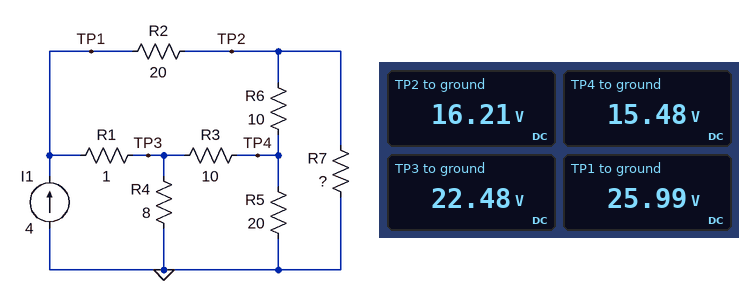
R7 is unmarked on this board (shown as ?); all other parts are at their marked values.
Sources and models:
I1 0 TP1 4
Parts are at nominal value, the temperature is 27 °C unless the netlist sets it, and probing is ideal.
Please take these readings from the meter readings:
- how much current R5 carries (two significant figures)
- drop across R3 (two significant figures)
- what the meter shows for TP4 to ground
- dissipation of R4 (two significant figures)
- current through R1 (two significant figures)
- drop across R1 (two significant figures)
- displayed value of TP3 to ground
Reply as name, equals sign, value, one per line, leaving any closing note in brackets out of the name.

how much current R5 carries = 770 mA
drop across R3 = 7.0 V
what the meter shows for TP4 to ground = 15.48 V
dissipation of R4 = 63 W
current through R1 = 3.5 A
drop across R1 = 3.5 V
displayed value of TP3 to ground = 22.48 V
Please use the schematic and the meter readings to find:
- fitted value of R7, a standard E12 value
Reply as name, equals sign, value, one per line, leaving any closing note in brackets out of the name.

fitted value of R7, a standard E12 value = 39 Ω
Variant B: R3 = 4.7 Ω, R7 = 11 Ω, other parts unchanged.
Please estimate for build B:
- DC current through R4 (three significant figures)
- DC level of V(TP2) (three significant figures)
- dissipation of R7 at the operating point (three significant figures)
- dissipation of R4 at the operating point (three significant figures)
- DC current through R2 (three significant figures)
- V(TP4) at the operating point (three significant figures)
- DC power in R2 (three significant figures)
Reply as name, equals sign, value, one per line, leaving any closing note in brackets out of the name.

DC current through R4 = 2.36 A
DC level of V(TP2) = 10.4 V
dissipation of R7 at the operating point = 9.84 W
dissipation of R4 at the operating point = 44.5 W
DC current through R2 = 593 mA
V(TP4) at the operating point = 13.9 V
DC power in R2 = 7.04 W
